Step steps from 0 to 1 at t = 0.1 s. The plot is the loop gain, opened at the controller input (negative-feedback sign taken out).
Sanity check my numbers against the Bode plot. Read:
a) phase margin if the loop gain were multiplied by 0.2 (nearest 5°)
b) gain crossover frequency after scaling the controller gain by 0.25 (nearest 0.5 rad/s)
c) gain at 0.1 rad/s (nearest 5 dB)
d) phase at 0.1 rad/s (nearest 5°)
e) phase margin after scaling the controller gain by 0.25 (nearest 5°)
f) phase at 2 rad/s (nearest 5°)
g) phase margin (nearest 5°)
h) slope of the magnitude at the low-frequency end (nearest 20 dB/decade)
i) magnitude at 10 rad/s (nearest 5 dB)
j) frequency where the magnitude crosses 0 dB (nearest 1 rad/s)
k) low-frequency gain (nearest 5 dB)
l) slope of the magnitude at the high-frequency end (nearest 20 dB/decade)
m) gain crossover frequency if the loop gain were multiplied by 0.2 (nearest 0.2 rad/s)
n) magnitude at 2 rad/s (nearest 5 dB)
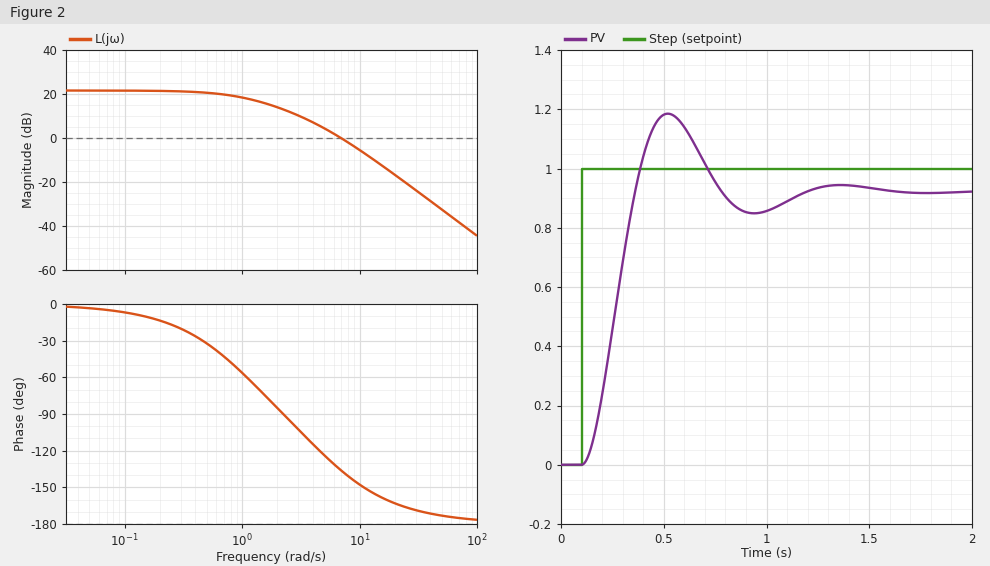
95°
2.5 rad/s
20 dB
-5°
85°
-85°
45°
0 dB/decade
-5 dB
7 rad/s
20 dB
-40 dB/decade
2.0 rad/s
15 dB
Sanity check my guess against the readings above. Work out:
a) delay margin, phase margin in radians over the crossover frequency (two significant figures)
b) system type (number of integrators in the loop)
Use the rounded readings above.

0.11 s
0
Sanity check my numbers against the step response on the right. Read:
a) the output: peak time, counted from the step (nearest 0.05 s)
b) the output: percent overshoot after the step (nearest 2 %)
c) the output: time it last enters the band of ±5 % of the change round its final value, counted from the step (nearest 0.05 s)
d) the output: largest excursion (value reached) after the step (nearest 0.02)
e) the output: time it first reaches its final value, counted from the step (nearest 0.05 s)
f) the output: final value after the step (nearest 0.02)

0.40 s
28 %
0.95 s
1.18
0.25 s
0.92
